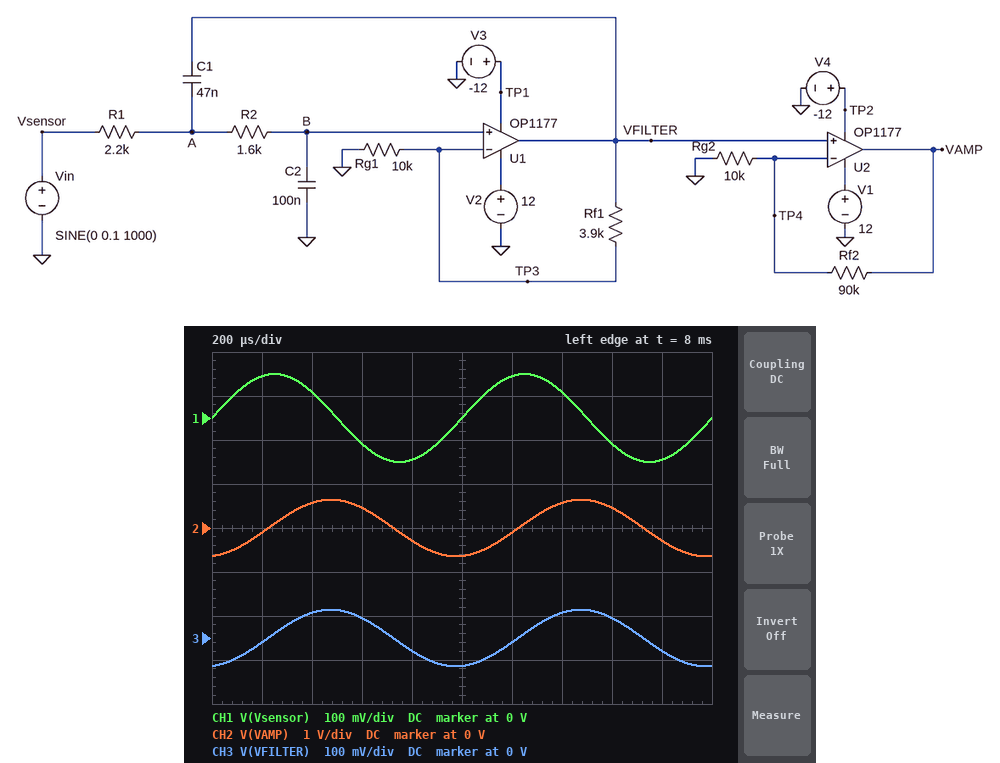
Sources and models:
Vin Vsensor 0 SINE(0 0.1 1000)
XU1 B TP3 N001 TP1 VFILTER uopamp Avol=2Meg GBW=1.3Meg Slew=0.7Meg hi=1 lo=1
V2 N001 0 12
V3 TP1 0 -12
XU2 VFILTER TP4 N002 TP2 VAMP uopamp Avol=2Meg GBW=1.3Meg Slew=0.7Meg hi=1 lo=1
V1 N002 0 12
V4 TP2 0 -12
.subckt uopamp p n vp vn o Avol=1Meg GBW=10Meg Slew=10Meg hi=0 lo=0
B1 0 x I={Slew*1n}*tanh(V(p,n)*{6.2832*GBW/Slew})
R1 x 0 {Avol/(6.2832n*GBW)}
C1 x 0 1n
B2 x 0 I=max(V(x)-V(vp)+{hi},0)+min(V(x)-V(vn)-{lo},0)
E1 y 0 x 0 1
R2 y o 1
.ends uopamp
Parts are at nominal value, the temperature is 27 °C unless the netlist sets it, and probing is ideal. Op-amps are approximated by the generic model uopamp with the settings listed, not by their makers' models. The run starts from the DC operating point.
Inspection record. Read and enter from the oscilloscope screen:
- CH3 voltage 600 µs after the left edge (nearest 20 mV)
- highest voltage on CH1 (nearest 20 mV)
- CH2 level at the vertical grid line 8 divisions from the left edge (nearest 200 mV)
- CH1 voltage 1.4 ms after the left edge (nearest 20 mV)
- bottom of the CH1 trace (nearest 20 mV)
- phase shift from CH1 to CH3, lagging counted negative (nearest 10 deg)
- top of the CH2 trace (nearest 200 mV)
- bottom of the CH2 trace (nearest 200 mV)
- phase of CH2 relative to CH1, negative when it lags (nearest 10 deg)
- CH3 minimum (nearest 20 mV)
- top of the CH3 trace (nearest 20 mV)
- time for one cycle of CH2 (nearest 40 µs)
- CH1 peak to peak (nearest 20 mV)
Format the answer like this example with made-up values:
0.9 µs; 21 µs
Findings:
40 mV; 100 mV; 400 mV; 60 mV; -100 mV; -80 deg; 600 mV; -600 mV; -80 deg; -60 mV; 60 mV; 1.00 ms; 200 mV
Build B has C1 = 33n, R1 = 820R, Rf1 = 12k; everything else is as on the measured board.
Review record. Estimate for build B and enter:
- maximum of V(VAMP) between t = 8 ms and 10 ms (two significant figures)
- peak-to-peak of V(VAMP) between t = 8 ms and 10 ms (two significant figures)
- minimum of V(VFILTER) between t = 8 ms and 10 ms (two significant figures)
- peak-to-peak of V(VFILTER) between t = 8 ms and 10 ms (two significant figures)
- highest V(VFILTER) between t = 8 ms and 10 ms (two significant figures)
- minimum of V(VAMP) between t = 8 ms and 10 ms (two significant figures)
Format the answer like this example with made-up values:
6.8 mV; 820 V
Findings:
1.4 V; 2.8 V; -140 mV; 280 mV; 140 mV; -1.4 V
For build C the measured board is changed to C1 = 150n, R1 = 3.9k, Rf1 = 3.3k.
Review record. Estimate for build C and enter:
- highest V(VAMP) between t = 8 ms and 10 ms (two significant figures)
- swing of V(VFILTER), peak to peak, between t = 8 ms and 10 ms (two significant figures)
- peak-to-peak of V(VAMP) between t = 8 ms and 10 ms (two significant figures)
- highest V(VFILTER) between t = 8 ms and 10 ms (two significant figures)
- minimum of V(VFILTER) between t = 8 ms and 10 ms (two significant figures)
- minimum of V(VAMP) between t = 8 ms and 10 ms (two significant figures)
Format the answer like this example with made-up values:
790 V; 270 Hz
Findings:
380 mV; 76 mV; 760 mV; 38 mV; -38 mV; -380 mV
